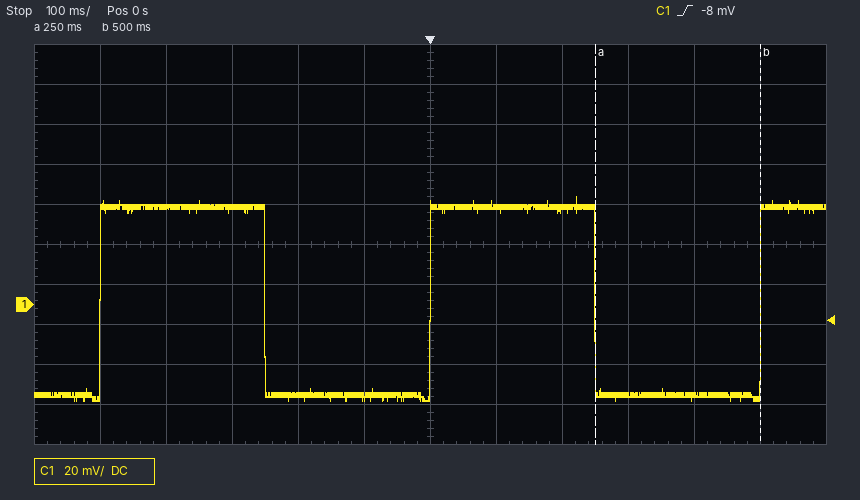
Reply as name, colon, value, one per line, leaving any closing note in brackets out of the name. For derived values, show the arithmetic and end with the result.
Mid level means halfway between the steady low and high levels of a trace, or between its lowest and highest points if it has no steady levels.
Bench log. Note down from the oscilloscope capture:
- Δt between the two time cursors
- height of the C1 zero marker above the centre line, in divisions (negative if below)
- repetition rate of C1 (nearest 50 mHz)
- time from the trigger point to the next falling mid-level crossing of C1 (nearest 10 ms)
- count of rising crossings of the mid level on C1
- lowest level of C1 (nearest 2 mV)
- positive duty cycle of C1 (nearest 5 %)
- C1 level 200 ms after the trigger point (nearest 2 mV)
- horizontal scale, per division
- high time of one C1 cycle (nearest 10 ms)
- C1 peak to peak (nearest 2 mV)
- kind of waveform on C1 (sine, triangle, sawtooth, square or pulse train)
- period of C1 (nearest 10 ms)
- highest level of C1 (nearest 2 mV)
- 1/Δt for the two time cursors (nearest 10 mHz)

Δt between the two time cursors: 500 ms − (250 ms) = 250 ms
height of the C1 zero marker above the centre line, in divisions: -1.5 div
repetition rate of C1: 1 / 500 ms ≈ 2.00 Hz
time from the trigger point to the next falling mid-level crossing of C1: 250 ms
count of rising crossings of the mid level on C1: 3
lowest level of C1: -48 mV
positive duty cycle of C1: 250 ms / 500 ms ≈ 50 %
C1 level 200 ms after the trigger point: 48 mV
horizontal scale, per division: 100 ms
high time of one C1 cycle: 250 ms
C1 peak to peak: 54 mV − (-48 mV) = 102 mV
kind of waveform on C1: square
period of C1: 500 ms
highest level of C1: 54 mV
1/Δt for the two time cursors: 1 / 250 ms ≈ 4.00 Hz
